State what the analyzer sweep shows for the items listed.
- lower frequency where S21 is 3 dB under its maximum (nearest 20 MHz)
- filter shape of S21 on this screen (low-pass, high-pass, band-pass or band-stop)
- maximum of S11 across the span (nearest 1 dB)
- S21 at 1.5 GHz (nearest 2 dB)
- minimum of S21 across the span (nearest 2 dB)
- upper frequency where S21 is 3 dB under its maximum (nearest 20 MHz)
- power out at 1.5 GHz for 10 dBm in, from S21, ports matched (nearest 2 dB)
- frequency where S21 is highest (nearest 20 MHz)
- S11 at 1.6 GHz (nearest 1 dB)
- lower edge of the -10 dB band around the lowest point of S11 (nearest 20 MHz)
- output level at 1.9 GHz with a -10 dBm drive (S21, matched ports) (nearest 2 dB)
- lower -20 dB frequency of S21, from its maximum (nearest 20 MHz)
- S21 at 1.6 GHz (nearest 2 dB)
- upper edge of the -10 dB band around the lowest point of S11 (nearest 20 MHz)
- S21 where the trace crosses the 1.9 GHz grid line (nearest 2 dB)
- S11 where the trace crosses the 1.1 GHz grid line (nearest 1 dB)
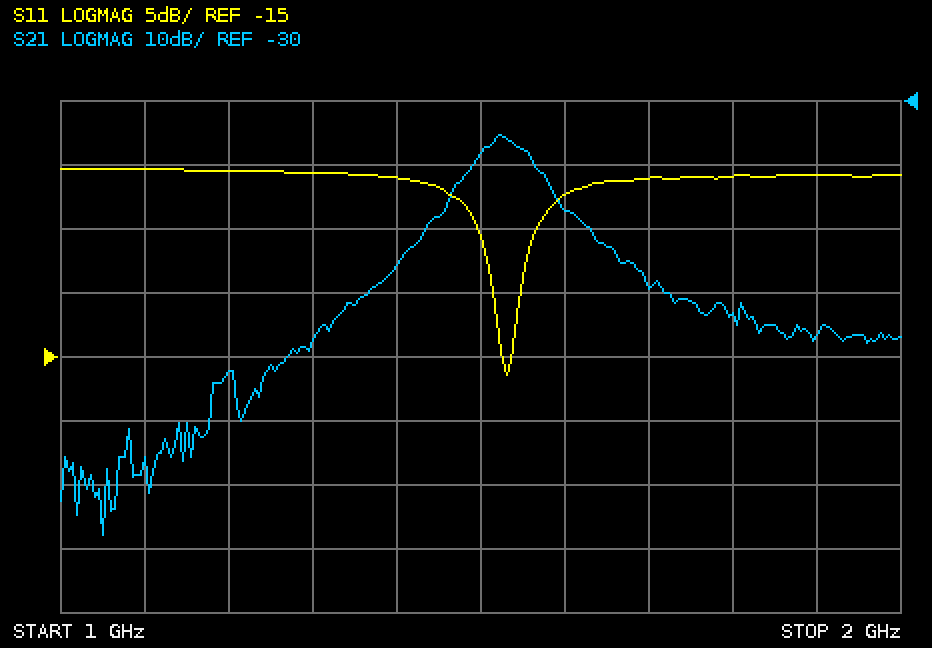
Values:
1.50 GHz
band-pass
0 dB
-38 dB
-98 dB
1.56 GHz
-28 dBm
1.52 GHz
-2 dB
1.52 GHz
-76 dBm
1.40 GHz
-48 dB
1.54 GHz
-66 dB
0 dB
